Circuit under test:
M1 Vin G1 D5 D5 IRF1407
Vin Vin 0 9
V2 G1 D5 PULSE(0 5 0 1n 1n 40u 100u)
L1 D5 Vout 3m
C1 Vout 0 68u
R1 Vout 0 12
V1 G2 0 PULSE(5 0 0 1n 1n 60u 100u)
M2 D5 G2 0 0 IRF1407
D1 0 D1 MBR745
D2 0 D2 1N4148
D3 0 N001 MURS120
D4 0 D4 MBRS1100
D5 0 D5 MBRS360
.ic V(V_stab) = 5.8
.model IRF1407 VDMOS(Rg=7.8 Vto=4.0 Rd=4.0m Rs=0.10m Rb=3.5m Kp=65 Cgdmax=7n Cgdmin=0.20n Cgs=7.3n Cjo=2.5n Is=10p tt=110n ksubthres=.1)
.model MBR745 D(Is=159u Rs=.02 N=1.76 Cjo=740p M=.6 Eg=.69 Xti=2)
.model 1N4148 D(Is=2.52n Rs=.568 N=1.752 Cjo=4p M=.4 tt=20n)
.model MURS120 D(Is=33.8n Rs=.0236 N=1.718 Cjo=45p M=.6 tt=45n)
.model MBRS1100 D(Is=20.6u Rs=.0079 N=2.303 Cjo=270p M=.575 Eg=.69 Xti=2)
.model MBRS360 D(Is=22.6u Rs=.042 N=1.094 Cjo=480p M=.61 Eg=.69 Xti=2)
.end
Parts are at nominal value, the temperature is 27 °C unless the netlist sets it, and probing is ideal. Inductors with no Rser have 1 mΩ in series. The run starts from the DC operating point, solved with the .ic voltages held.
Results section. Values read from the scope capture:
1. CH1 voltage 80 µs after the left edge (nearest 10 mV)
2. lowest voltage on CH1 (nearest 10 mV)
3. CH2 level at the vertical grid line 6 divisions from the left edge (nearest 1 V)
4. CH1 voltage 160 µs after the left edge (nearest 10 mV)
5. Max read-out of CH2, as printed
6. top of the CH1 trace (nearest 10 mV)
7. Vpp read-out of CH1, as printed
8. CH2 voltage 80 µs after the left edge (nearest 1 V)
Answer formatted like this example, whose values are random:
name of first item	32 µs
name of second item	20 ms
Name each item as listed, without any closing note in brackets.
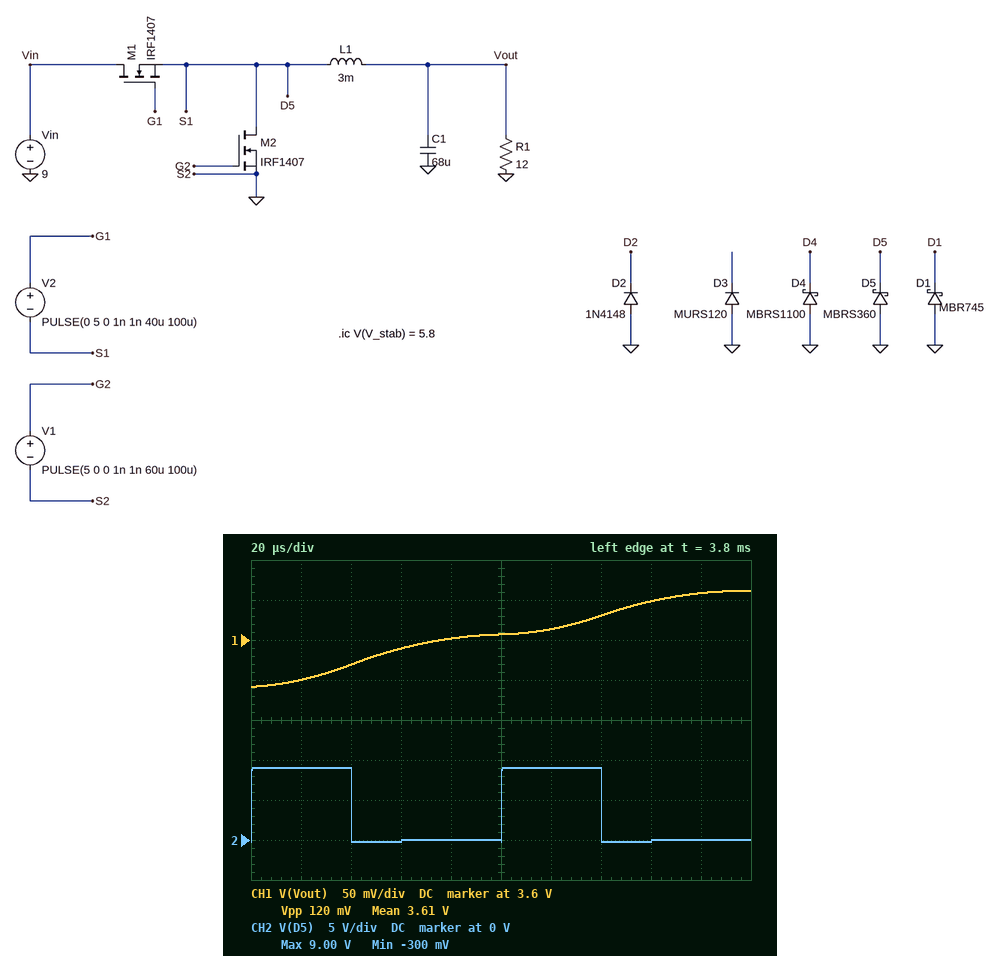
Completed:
CH1 voltage 80 µs after the left edge	3.60 V
lowest voltage on CH1	3.54 V
CH2 level at the vertical grid line 6 divisions from the left edge	9 V
CH1 voltage 160 µs after the left edge	3.65 V
Max read-out of CH2, as printed	9.00 V
top of the CH1 trace	3.66 V
Vpp read-out of CH1, as printed	120 mV
CH2 voltage 80 µs after the left edge	0 V
